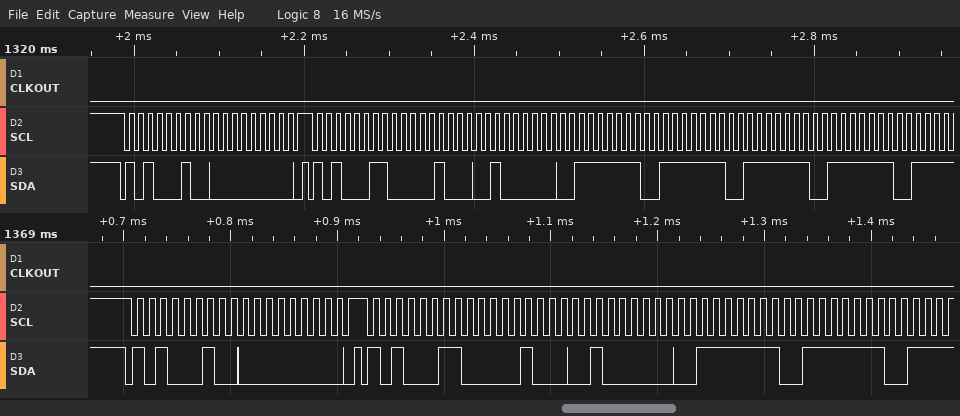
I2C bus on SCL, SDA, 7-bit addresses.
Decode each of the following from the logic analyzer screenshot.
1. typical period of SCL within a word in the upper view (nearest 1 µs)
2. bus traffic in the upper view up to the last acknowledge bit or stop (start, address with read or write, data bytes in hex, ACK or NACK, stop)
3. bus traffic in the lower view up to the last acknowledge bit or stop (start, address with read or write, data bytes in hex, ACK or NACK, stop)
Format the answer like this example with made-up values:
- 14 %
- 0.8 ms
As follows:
- 11 µs
- start, address 51 write ACK, 00 ACK, stop, start, address 51 read ACK, 08 ACK, 40 ACK, 7F ACK, 7F ACK, 7F ACK, 7F ACK
- start, address 51 write ACK, 00 ACK, stop, start, address 51 read ACK, 08 ACK, 40 ACK, 7F ACK, 7F ACK
